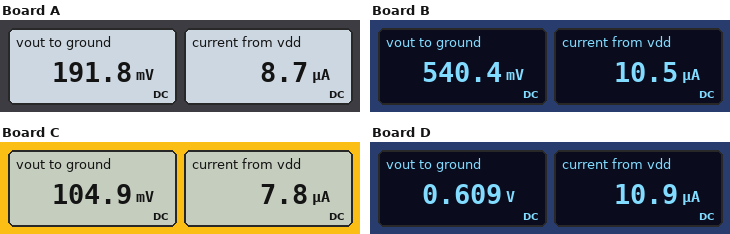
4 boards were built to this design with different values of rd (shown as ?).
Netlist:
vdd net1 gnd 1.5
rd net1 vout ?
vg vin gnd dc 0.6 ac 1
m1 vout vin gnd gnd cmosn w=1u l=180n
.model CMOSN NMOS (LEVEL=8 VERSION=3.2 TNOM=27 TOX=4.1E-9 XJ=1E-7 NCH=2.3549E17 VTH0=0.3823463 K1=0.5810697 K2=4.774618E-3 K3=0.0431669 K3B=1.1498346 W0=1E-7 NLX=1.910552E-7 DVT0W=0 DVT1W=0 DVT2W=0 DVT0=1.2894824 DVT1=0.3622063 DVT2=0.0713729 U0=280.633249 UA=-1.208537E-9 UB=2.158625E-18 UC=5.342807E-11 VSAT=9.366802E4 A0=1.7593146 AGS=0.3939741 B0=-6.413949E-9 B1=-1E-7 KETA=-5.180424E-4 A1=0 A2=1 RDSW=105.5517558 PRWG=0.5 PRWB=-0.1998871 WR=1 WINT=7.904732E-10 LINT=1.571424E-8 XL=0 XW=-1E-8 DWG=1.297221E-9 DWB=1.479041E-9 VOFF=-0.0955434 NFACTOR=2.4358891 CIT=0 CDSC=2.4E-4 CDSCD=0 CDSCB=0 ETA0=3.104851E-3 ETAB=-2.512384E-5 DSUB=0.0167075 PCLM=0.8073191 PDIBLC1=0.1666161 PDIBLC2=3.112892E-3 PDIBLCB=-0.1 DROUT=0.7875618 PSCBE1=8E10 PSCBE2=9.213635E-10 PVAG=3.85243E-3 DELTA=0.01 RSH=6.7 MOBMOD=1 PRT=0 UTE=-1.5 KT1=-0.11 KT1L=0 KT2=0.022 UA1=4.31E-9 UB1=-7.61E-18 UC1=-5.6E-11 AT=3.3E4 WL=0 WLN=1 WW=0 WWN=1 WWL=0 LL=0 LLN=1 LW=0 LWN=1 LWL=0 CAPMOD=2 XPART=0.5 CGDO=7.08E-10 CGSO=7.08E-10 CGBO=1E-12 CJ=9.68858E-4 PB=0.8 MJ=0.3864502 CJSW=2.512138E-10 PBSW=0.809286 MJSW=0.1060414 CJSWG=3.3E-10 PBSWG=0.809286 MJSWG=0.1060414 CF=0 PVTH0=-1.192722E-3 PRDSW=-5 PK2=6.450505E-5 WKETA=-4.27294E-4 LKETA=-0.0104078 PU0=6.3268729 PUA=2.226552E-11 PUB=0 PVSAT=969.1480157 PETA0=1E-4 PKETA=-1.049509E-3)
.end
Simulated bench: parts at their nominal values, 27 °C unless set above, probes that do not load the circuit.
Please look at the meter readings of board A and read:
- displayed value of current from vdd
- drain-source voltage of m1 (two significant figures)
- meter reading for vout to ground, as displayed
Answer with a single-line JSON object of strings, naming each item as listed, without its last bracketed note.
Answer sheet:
{"displayed value of current from vdd": "8.7 µA", "drain-source voltage of m1": "190 mV", "meter reading for vout to ground, as displayed": "191.8 mV"}
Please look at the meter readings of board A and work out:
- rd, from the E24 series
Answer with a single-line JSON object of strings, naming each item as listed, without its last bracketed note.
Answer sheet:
{"rd, from the E24 series": "150 kΩ"}
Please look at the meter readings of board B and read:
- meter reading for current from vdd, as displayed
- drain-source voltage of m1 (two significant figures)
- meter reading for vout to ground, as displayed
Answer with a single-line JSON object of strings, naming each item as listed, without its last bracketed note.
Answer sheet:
{"meter reading for current from vdd, as displayed": "10.5 µA", "drain-source voltage of m1": "540 mV", "meter reading for vout to ground, as displayed": "540.4 mV"}
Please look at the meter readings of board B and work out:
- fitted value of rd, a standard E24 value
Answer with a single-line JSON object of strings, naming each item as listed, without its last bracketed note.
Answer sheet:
{"fitted value of rd, a standard E24 value": "91 kΩ"}
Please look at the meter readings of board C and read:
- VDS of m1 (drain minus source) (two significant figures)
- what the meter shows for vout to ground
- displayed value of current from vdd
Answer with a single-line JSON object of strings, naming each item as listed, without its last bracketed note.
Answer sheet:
{"VDS of m1 (drain minus source)": "100 mV", "what the meter shows for vout to ground": "104.9 mV", "displayed value of current from vdd": "7.8 µA"}
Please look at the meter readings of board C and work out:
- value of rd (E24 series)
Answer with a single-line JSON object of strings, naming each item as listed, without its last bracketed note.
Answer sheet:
{"value of rd": "180 kΩ"}
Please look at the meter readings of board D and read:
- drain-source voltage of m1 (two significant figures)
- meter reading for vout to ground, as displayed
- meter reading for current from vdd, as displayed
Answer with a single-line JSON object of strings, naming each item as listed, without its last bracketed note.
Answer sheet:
{"drain-source voltage of m1": "610 mV", "meter reading for vout to ground, as displayed": "0.609 V", "meter reading for current from vdd, as displayed": "10.9 µA"}
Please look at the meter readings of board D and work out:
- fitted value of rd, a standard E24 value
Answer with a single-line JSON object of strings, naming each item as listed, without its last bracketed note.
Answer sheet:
{"fitted value of rd, a standard E24 value": "82 kΩ"}
